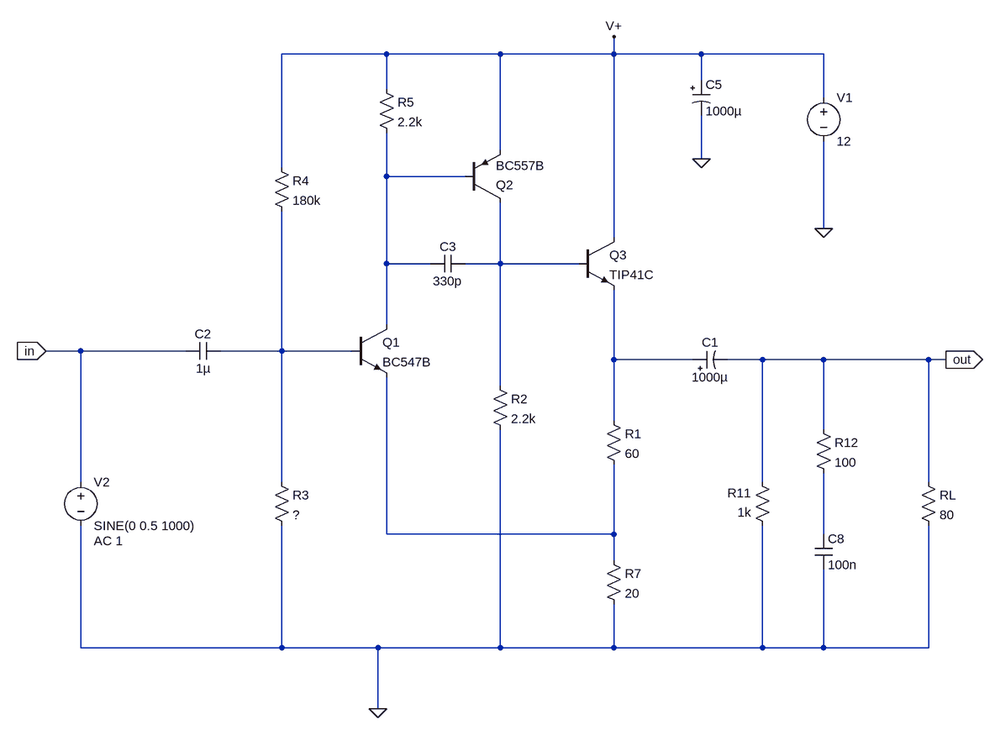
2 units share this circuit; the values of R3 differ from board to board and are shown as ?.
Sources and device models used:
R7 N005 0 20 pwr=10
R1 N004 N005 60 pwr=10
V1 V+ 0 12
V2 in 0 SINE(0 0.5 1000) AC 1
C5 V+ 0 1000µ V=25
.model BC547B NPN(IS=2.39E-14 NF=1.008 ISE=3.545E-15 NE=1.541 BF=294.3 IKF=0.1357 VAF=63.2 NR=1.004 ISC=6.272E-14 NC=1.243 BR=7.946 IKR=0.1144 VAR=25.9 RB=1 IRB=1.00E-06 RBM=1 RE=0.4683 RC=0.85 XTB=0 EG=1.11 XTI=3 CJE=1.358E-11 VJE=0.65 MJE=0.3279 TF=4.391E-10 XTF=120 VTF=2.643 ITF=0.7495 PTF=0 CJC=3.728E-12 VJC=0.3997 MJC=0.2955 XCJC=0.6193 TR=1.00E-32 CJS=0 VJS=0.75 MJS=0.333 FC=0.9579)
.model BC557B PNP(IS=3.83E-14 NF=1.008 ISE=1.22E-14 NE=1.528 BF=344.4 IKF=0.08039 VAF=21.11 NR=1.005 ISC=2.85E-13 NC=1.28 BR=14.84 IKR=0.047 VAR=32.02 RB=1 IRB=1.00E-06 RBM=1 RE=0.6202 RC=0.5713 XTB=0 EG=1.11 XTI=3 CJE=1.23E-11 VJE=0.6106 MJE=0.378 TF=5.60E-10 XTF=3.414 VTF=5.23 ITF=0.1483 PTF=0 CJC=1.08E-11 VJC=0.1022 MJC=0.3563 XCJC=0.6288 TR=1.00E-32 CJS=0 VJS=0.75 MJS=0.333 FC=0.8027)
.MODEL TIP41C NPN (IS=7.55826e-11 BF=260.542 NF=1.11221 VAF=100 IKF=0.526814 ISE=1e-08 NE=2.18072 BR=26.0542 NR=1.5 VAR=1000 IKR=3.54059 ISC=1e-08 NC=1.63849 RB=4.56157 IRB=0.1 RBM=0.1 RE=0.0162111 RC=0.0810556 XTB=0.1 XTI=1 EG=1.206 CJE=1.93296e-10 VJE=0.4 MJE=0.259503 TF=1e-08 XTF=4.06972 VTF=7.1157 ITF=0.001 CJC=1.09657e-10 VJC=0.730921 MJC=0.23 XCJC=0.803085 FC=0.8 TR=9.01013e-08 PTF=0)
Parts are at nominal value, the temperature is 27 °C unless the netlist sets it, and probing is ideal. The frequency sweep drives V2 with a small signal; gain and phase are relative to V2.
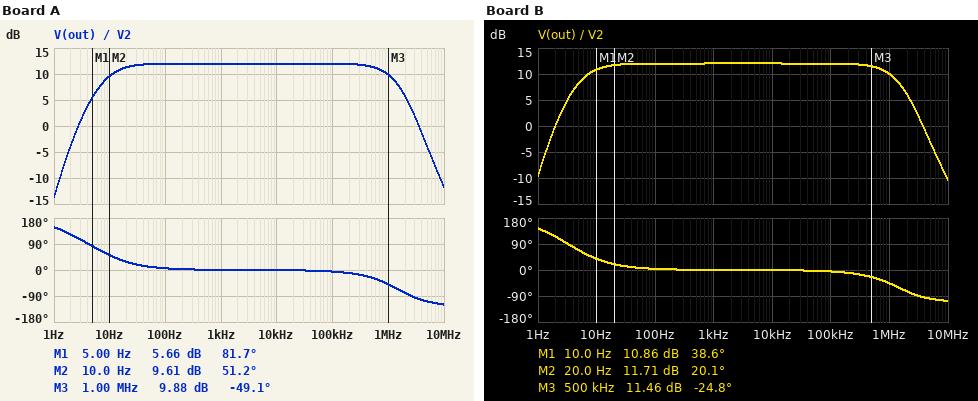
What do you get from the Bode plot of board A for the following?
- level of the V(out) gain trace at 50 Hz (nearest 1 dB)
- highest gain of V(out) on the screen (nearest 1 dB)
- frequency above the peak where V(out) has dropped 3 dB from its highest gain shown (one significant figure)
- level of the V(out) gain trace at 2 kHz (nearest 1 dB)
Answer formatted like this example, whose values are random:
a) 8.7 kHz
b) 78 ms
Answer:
a) 12 dB
b) 12 dB
c) 1 MHz
d) 12 dB
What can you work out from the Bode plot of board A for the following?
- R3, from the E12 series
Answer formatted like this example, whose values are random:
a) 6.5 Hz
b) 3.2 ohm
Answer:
a) 22 kΩ
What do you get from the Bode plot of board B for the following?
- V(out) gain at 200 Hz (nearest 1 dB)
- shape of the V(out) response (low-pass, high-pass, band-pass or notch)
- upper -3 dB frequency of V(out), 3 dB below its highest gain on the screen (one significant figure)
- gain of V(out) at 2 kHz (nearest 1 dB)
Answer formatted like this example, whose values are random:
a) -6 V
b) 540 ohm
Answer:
a) 12 dB
b) band-pass
c) 1 MHz
d) 12 dB
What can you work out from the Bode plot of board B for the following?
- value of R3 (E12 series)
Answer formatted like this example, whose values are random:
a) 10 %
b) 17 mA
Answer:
a) 39 kΩ
